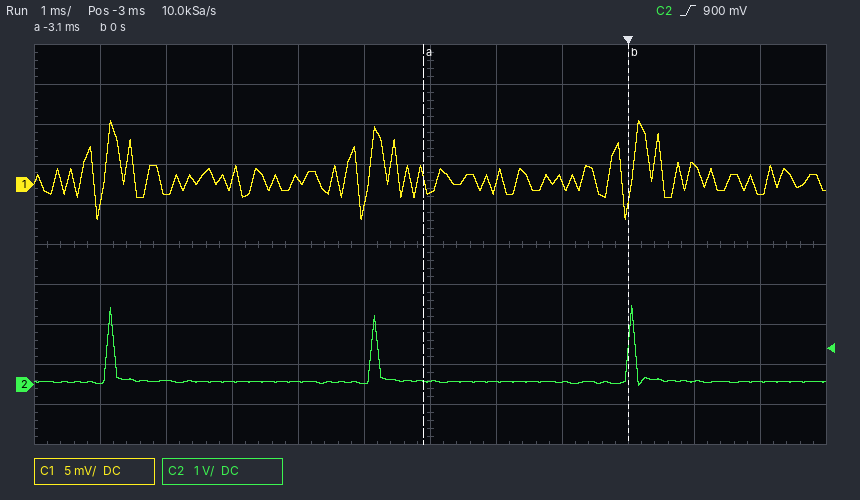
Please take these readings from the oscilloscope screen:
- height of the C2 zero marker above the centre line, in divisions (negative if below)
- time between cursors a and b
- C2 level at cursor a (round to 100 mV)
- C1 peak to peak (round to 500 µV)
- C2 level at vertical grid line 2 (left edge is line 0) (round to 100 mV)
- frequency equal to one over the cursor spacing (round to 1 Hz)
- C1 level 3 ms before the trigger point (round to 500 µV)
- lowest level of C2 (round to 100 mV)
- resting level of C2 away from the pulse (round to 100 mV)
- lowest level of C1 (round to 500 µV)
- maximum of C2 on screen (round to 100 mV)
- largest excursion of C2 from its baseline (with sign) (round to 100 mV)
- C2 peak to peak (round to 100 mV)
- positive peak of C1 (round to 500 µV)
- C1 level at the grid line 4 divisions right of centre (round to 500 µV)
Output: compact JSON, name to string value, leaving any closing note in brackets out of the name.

{"height of the C2 zero marker above the centre line, in divisions": "-3.5 div", "time between cursors a and b": "3.1 ms", "C2 level at cursor a": "100 mV", "C1 peak to peak": "12.5 mV", "C2 level at vertical grid line 2 (left edge is line 0)": "100 mV", "frequency equal to one over the cursor spacing": "323 Hz", "C1 level 3 ms before the trigger point": "-1.0 mV", "lowest level of C2": "0.0 V", "resting level of C2 away from the pulse": "100 mV", "lowest level of C1": "-4.5 mV", "maximum of C2 on screen": "2.0 V", "largest excursion of C2 from its baseline (with sign)": "+1.9 V", "C2 peak to peak": "2.0 V", "positive peak of C1": "8.0 mV", "C1 level at the grid line 4 divisions right of centre": "2.5 mV"}
